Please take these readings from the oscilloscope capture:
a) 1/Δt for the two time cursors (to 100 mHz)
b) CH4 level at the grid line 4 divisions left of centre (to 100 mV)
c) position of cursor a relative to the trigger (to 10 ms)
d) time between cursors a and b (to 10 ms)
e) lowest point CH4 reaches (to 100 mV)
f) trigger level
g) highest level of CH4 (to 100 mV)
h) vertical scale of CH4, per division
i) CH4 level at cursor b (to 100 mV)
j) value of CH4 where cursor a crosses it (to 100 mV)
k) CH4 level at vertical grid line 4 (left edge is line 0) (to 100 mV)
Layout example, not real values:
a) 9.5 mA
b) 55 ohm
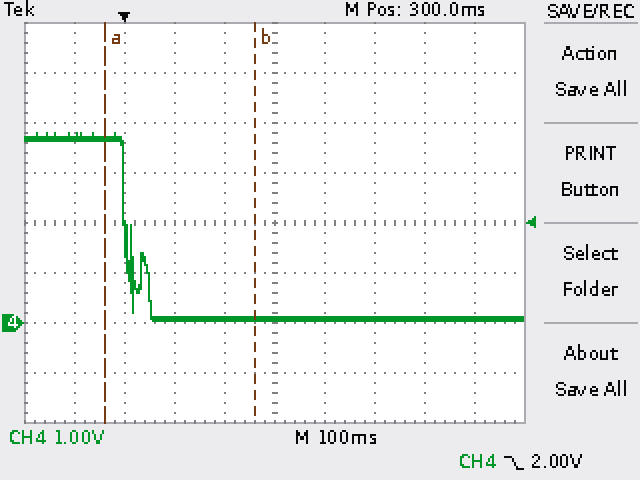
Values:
a) 3.3 Hz
b) 3.7 V
c) -40 ms
d) 300 ms
e) 0.0 V
f) 2.00 V
g) 3.8 V
h) 1 V
i) 100 mV
j) 3.7 V
k) 100 mV
